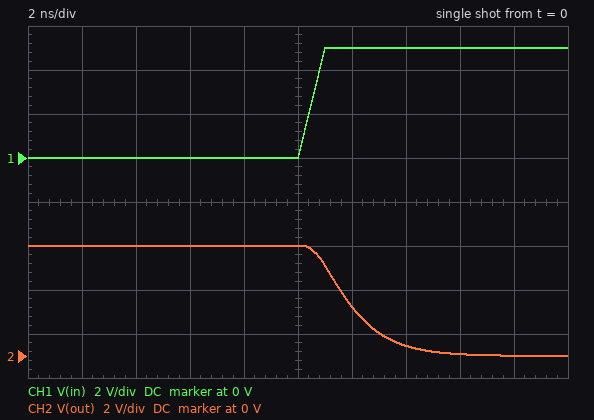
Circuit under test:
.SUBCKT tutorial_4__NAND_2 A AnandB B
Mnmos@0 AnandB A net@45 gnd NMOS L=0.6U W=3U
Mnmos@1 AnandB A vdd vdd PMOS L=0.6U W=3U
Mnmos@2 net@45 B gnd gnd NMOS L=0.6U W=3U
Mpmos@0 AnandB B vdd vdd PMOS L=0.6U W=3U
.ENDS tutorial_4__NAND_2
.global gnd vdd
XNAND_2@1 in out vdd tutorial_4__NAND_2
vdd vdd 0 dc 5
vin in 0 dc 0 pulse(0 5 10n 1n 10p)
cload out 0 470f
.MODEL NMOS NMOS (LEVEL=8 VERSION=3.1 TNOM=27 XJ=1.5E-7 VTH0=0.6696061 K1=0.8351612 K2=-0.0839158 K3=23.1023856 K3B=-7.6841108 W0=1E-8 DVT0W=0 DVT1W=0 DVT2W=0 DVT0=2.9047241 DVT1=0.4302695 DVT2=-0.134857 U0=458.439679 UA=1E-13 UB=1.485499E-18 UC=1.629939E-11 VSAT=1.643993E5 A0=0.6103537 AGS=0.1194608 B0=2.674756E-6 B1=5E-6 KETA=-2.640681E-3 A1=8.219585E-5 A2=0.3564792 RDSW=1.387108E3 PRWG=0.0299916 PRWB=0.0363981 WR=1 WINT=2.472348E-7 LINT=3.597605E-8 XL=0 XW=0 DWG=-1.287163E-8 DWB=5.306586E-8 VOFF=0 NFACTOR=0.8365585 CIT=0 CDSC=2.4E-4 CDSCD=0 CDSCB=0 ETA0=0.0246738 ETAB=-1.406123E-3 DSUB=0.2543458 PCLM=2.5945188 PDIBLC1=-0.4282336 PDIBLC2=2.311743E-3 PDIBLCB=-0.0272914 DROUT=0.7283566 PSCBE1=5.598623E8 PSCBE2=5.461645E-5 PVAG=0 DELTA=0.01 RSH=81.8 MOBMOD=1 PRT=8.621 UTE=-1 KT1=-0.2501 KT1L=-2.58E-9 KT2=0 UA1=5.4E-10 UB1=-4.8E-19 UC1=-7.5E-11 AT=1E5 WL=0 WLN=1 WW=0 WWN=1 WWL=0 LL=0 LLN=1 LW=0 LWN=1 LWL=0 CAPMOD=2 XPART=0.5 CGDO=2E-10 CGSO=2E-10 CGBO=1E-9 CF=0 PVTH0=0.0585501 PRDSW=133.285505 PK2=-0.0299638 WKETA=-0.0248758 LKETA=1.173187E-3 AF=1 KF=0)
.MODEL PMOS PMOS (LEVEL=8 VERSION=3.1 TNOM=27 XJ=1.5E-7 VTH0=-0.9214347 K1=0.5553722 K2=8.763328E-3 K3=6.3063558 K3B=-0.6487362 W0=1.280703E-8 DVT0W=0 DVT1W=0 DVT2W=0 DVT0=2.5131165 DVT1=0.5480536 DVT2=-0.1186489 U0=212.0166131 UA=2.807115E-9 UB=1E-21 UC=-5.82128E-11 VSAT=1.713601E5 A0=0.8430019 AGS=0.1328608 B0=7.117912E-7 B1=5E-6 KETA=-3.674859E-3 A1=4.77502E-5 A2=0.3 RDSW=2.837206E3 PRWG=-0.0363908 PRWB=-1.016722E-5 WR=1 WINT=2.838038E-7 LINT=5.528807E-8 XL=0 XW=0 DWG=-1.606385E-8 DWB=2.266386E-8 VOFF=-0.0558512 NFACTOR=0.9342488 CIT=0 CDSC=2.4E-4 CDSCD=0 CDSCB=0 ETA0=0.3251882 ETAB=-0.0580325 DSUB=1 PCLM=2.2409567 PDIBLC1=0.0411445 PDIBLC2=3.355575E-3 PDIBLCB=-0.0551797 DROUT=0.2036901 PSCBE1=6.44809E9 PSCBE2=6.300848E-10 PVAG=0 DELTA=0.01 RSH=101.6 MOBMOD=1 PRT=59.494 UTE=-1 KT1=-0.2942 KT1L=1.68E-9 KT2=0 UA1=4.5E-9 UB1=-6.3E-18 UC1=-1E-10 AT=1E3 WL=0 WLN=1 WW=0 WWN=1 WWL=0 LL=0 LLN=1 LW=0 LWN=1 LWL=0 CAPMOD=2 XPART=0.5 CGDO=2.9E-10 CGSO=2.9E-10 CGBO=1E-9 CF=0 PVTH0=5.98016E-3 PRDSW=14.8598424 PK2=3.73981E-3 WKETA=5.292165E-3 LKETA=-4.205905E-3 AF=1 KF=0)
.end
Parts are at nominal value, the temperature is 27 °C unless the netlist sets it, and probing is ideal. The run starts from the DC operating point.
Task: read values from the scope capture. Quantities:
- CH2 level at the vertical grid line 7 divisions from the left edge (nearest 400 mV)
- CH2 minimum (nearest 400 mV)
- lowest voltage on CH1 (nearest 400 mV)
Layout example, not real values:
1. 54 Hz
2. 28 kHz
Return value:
1. 400 mV
2. 0 V
3. 0 V
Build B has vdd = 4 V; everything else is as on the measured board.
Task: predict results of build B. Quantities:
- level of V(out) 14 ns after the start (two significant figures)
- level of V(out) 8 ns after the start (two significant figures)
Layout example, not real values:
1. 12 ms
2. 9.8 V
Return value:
1. 330 mV
2. 4.0 V
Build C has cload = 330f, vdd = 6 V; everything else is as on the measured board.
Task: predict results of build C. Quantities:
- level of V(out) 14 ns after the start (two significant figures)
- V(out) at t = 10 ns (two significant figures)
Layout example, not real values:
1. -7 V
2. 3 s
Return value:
1. 210 mV
2. 6.0 V
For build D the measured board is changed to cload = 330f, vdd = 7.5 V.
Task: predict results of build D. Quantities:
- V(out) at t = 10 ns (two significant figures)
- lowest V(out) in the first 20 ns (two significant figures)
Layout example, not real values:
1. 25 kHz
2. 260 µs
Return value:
1. 7.5 V
2. 710 mV
